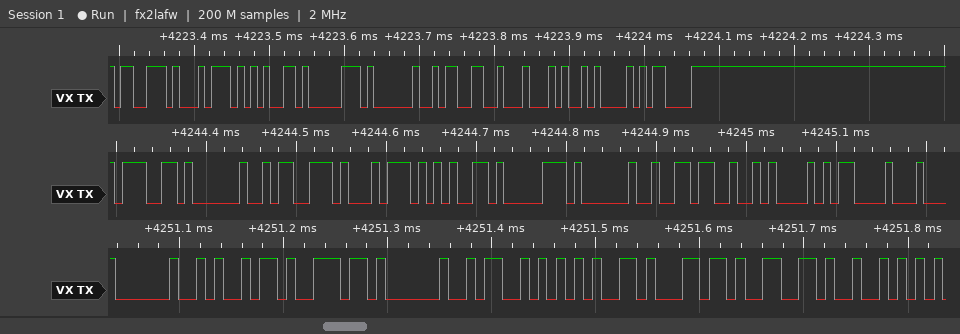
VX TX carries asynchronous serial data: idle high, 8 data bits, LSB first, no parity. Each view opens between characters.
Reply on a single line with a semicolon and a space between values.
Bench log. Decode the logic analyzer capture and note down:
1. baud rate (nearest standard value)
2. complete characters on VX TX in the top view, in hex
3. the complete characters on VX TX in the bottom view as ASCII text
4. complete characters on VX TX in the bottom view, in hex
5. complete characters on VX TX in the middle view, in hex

115200 baud; 73, 74, 65, 70, 20, 33, 44, 0A, 0D; " in SelfR"; 20, 69, 6E, 20, 53, 65, 6C, 66, 52; 67, 20, 73, 74, 65, 70, 20, 36, 0A, 0D
